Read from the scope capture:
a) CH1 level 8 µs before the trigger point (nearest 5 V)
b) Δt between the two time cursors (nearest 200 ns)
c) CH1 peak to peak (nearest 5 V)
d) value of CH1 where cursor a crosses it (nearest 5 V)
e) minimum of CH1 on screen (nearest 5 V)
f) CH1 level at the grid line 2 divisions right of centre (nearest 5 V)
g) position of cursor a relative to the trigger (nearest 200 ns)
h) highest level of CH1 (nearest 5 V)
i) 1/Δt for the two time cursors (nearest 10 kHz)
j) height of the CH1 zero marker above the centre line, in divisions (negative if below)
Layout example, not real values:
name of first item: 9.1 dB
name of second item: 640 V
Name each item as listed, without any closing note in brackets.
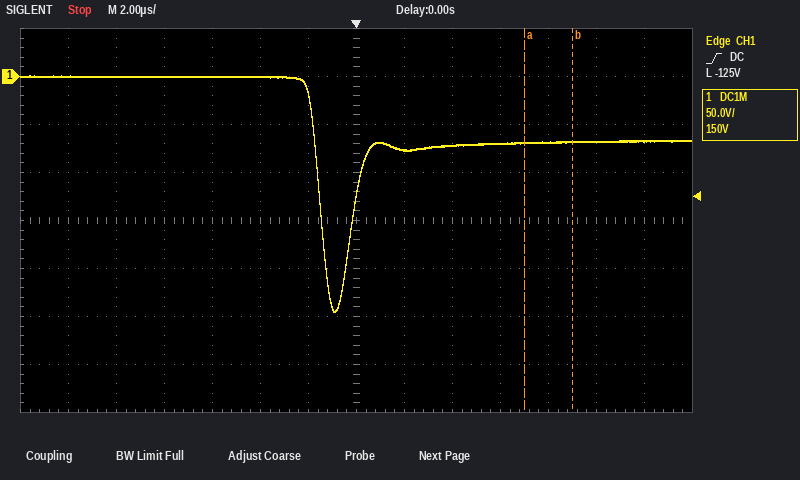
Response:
CH1 level 8 µs before the trigger point: 0 V
Δt between the two time cursors: 2.0 µs
CH1 peak to peak: 245 V
value of CH1 where cursor a crosses it: -70 V
minimum of CH1 on screen: -245 V
CH1 level at the grid line 2 divisions right of centre: -70 V
position of cursor a relative to the trigger: +7.0 µs
highest level of CH1: 0 V
1/Δt for the two time cursors: 500 kHz
height of the CH1 zero marker above the centre line, in divisions: +3.0 div
